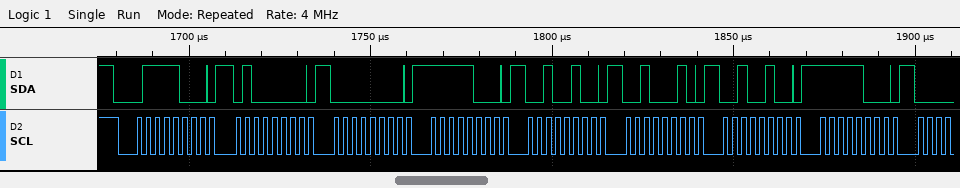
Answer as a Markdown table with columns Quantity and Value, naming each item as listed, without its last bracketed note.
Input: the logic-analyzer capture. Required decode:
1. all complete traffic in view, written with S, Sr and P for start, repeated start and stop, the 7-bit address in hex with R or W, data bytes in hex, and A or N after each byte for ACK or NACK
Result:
| Quantity | Value |
|---|---|
| all complete traffic in view, written with S, Sr and P for start, repeated start and stop, the 7-bit address in hex with R or W, data bytes in hex, and A or N after each byte for ACK or NACK | S 3CW A 40 A 00 A F8 A 24 A 22 A 24 A F8 A |
